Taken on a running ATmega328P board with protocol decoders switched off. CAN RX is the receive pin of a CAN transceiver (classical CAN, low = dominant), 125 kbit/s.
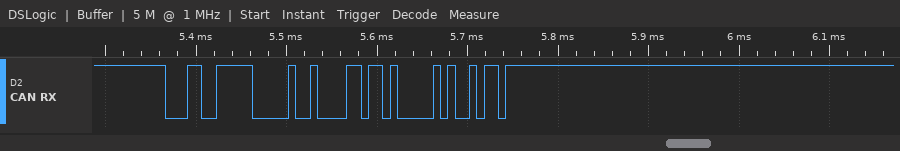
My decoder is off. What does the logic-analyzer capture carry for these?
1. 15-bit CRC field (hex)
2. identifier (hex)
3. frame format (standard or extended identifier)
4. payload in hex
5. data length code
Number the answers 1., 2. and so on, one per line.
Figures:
1. 0x5025
2. 0x19F
3. standard
4. 0D
5. 1
